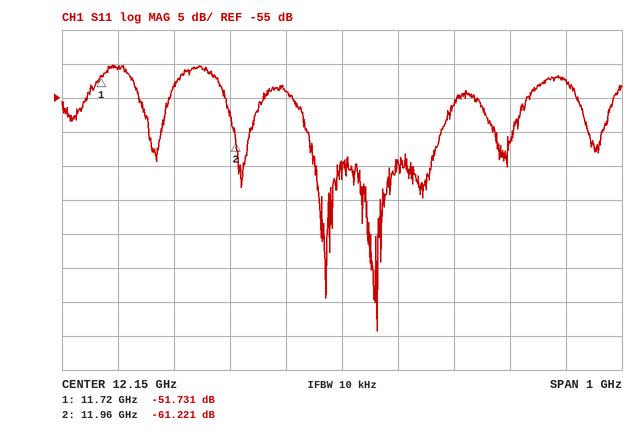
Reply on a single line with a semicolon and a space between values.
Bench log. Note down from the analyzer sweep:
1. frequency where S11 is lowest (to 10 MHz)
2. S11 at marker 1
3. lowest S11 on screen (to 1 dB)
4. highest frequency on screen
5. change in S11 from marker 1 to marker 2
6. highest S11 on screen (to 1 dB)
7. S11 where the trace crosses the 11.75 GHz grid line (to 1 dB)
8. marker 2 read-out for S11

12.21 GHz; -51.731 dB; -89 dB; 12.65 GHz; -9.490 dB; -50 dB; -51 dB; -61.221 dB
